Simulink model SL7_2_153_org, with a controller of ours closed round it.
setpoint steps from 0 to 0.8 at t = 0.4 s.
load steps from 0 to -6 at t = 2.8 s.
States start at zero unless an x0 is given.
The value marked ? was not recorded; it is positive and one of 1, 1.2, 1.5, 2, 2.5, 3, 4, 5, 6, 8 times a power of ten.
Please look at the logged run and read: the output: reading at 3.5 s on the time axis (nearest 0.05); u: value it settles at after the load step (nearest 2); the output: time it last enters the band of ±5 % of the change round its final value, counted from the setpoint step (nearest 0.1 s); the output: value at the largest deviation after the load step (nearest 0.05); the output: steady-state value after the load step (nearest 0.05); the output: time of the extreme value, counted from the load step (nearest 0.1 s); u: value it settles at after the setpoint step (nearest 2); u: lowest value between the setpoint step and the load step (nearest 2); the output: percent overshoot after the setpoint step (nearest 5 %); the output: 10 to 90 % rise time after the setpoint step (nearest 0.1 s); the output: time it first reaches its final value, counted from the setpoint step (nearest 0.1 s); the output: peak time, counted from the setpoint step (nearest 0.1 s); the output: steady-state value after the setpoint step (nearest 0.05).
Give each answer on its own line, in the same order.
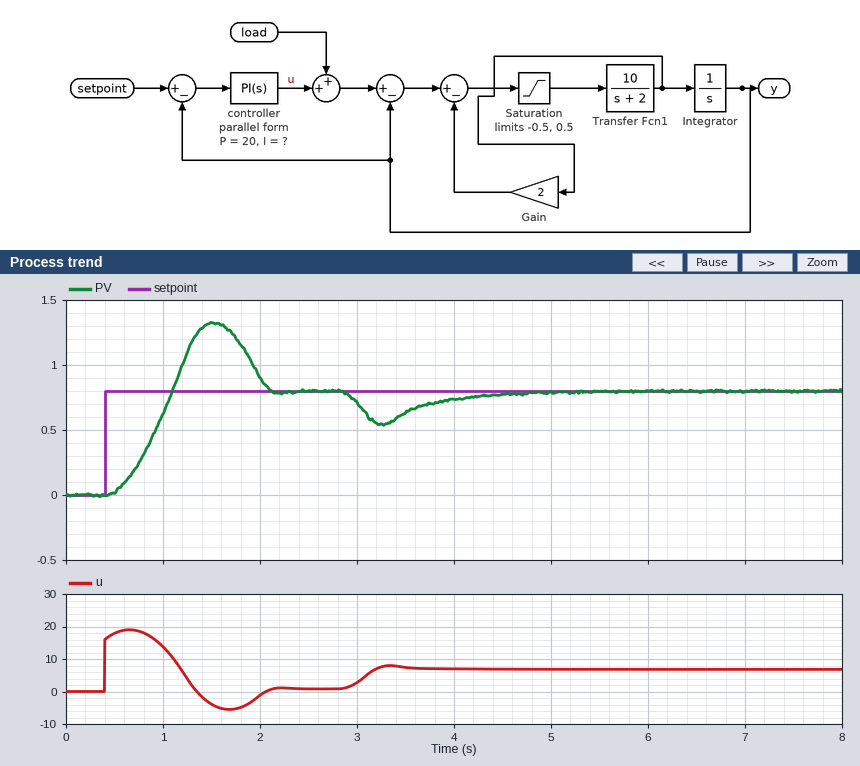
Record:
0.65
6
1.7 s
0.55
0.80
0.5 s
0
-6
65 %
0.5 s
0.7 s
1.1 s
0.80
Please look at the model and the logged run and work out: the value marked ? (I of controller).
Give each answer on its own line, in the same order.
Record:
30
